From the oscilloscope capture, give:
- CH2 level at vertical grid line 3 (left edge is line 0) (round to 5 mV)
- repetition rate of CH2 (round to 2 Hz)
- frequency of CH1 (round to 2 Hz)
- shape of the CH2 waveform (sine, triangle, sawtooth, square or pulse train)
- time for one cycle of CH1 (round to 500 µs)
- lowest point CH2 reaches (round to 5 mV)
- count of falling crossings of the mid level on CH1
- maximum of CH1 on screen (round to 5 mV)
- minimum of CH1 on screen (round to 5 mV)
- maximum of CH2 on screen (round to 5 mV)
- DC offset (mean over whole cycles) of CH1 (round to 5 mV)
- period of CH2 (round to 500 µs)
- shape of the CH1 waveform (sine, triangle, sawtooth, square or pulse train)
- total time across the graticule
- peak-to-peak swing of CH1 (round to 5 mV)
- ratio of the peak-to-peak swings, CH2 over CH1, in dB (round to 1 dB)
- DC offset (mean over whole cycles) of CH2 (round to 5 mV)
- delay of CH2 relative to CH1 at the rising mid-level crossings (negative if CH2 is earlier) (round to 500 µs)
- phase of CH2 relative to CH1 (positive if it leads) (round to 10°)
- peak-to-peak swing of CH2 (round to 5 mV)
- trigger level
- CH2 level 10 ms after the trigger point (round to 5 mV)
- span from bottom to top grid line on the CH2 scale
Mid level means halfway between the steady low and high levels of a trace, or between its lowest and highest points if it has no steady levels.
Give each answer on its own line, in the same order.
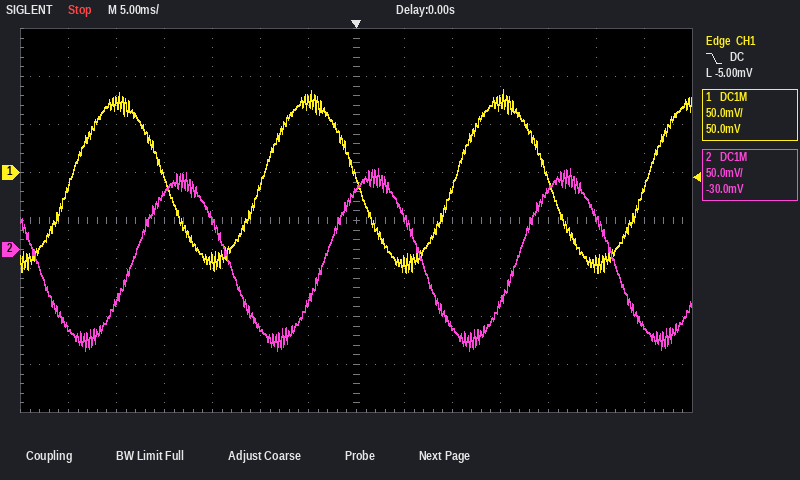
60 mV
50 Hz
50 Hz
sine
20.0 ms
-105 mV
3
85 mV
-105 mV
85 mV
-10 mV
20.0 ms
sine
70 ms
190 mV
0 dB
-10 mV
+6.5 ms
-120°
190 mV
-5.00 mV
-80 mV
400 mV
